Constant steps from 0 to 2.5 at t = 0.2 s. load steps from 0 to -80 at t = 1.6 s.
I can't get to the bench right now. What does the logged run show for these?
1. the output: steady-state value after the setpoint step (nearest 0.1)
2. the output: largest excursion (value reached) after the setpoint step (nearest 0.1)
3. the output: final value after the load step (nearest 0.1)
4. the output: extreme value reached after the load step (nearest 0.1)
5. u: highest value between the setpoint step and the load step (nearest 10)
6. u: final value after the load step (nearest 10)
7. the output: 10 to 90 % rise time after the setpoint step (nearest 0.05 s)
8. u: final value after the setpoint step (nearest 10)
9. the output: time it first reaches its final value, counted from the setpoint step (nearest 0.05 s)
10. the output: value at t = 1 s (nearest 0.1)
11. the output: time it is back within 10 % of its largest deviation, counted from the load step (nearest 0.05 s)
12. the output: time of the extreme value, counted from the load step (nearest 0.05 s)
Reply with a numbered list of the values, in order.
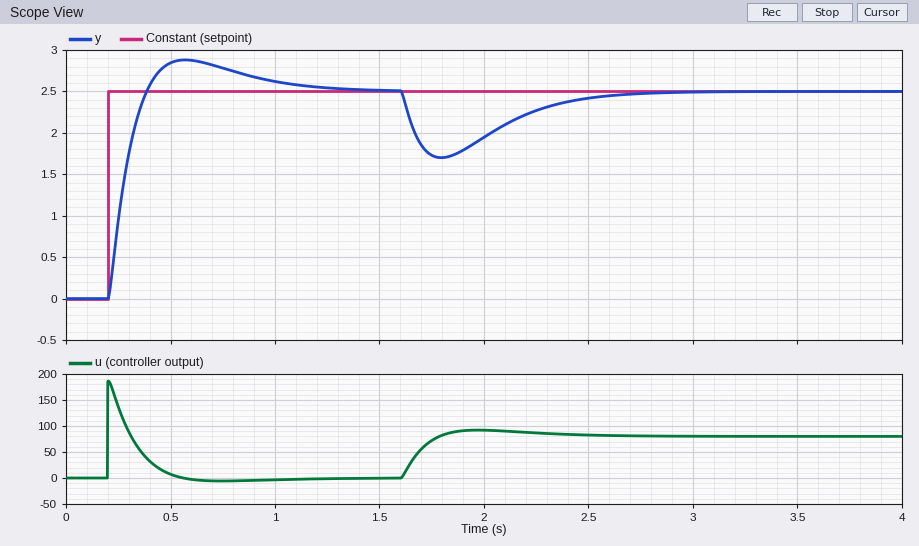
1. 2.5
2. 2.9
3. 2.5
4. 1.7
5. 190
6. 80
7. 0.15 s
8. 0
9. 0.20 s
10. 2.6
11. 0.90 s
12. 0.20 s
